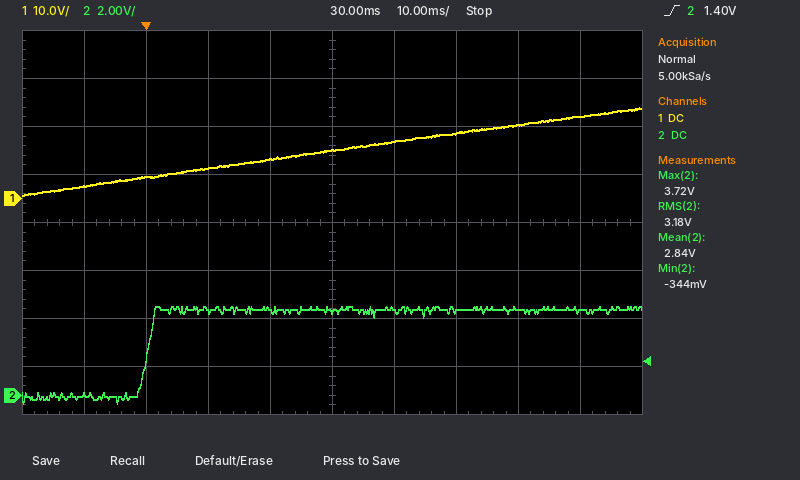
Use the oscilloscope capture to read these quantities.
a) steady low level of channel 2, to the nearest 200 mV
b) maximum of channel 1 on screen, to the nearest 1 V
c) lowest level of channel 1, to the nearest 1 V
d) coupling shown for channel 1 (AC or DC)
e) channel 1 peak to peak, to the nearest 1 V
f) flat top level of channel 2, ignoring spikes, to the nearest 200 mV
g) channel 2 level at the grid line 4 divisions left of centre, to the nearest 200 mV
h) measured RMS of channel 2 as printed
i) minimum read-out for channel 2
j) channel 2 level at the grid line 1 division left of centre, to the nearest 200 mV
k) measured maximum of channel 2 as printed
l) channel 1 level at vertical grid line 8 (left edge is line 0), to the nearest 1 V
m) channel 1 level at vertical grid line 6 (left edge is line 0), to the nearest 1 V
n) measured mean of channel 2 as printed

0.0 V
19 V
1 V
DC
18 V
3.6 V
0.0 V
3.18 V
-344 mV
3.6 V
3.72 V
15 V
12 V
2.84 V
